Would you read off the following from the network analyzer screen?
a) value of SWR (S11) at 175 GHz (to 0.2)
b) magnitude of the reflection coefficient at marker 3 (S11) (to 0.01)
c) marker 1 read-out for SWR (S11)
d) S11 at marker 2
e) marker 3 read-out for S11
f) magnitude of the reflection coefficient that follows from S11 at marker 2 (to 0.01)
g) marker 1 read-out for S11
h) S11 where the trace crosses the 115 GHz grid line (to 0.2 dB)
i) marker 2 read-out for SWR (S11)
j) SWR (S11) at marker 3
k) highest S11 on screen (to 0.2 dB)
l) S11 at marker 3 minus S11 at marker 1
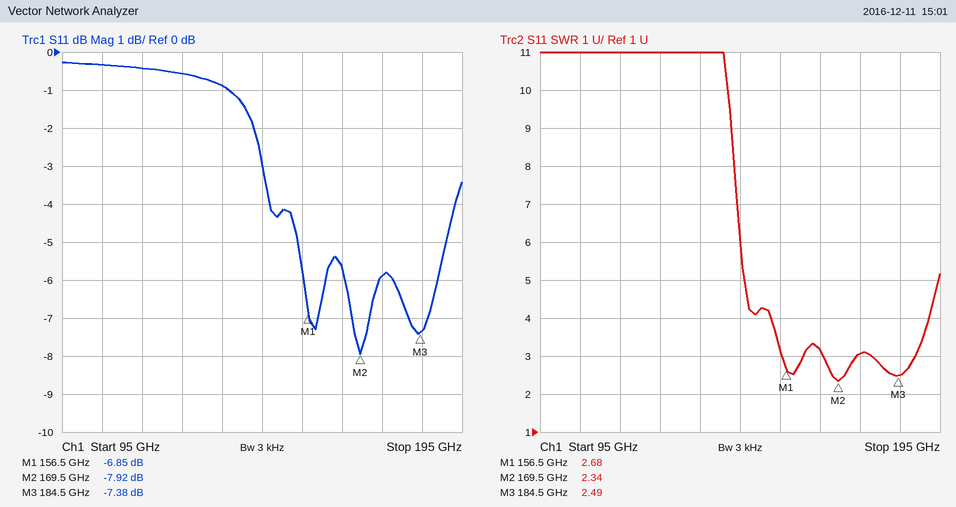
3.0
0.43
2.68
-7.92 dB
-7.38 dB
0.40
-6.85 dB
-0.4 dB
2.34
2.49
-0.2 dB
-0.53 dB
